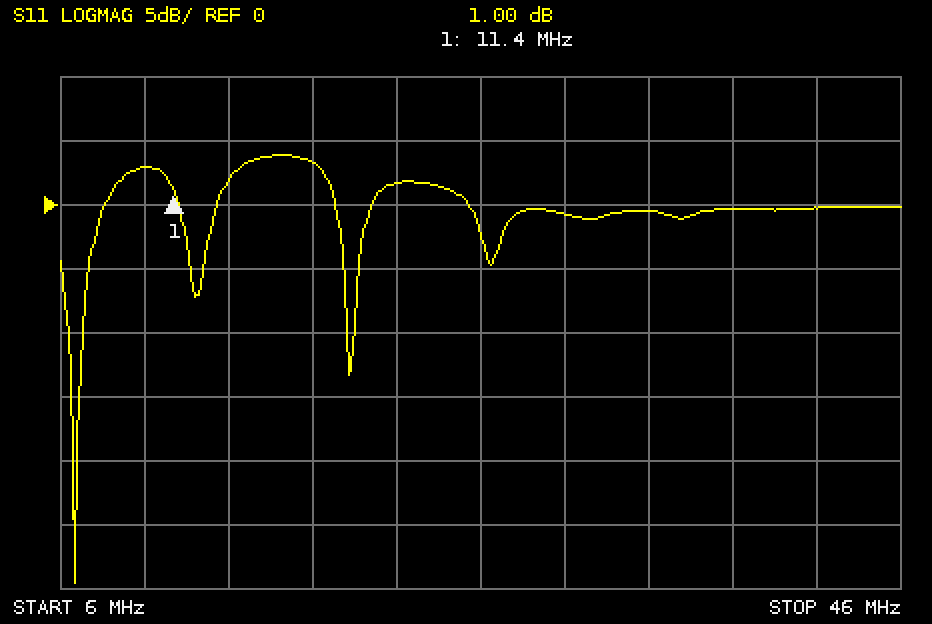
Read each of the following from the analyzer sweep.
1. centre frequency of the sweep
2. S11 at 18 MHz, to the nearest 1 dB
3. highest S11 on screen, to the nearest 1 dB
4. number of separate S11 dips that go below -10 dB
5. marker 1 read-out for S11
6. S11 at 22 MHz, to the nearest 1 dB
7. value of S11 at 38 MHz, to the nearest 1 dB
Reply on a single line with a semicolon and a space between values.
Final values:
26 MHz; 3 dB; 4 dB; 2; 1.00 dB; 2 dB; 0 dB
